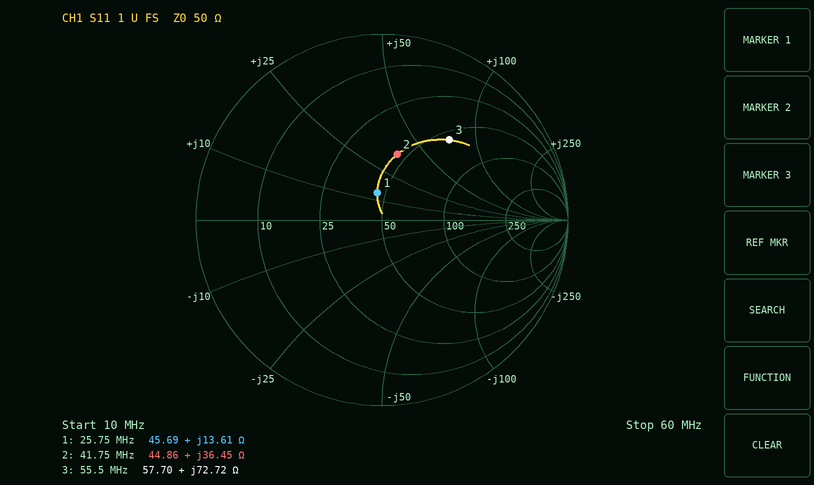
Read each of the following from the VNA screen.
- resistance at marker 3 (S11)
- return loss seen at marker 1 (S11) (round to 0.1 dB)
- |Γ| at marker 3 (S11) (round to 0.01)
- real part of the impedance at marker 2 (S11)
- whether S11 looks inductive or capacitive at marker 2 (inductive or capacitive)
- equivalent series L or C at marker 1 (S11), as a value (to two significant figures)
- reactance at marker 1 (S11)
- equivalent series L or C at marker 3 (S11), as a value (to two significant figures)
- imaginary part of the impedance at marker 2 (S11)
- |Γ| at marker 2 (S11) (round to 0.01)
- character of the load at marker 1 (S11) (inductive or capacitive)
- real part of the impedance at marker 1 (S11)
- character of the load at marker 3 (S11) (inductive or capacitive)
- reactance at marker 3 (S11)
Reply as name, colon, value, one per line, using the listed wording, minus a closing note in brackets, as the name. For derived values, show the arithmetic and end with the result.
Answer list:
resistance at marker 3: 57.70 Ω
return loss seen at marker 1 (S11): 16.6 dB
|Γ| at marker 3 (S11): 0.56
real part of the impedance at marker 2: 44.86 Ω
whether S11 looks inductive or capacitive at marker 2: inductive
equivalent series L or C at marker 1 (S11), as a value: L = 13.61 Ω/(2π × 25.75 MHz) ≈ 84 nH
reactance at marker 1: +13.61 Ω
equivalent series L or C at marker 3 (S11), as a value: L = 72.72 Ω/(2π × 55.5 MHz) ≈ 209 nH, so 210 nH to two significant figures
imaginary part of the impedance at marker 2: +36.45 Ω
|Γ| at marker 2 (S11): 0.36
character of the load at marker 1 (S11): inductive
real part of the impedance at marker 1: 45.69 Ω
character of the load at marker 3 (S11): inductive
reactance at marker 3: +72.72 Ω
